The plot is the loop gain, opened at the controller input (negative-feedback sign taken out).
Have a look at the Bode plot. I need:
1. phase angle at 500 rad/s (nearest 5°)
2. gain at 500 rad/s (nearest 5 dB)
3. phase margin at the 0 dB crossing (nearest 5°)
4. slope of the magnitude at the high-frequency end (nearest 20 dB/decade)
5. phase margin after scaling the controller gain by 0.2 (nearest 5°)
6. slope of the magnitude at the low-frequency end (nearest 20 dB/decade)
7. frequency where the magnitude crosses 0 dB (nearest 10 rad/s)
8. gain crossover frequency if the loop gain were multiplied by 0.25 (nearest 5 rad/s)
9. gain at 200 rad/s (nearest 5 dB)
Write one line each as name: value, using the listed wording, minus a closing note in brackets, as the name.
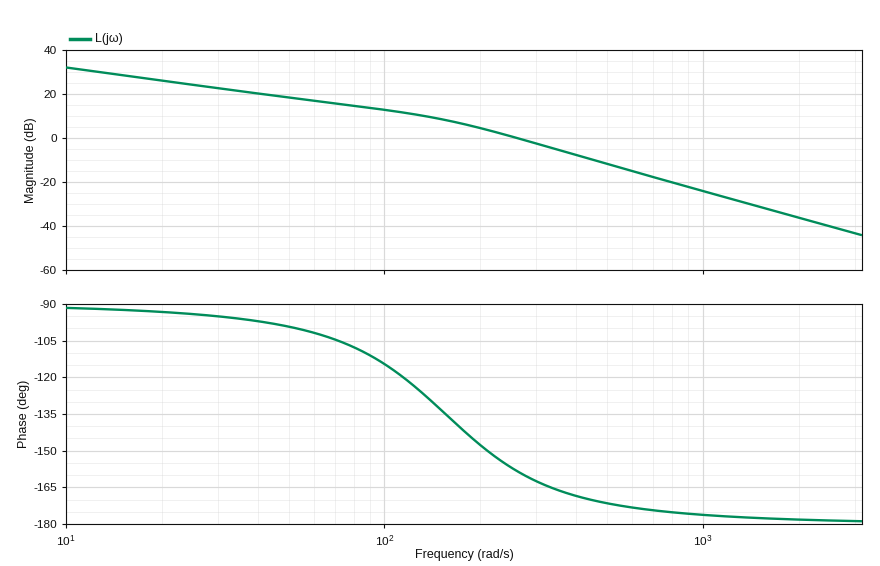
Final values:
phase angle at 500 rad/s: -170°
gain at 500 rad/s: -10 dB
phase margin at the 0 dB crossing: 20°
slope of the magnitude at the high-frequency end: -40 dB/decade
phase margin after scaling the controller gain by 0.2: 70°
slope of the magnitude at the low-frequency end: -20 dB/decade
frequency where the magnitude crosses 0 dB: 260 rad/s
gain crossover frequency if the loop gain were multiplied by 0.25: 110 rad/s
gain at 200 rad/s: 5 dB
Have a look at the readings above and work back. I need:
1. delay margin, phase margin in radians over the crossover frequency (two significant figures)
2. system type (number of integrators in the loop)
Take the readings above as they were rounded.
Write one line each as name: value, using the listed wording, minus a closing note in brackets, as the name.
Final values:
delay margin, phase margin in radians over the crossover frequency: 0.0013 s
system type: 1
